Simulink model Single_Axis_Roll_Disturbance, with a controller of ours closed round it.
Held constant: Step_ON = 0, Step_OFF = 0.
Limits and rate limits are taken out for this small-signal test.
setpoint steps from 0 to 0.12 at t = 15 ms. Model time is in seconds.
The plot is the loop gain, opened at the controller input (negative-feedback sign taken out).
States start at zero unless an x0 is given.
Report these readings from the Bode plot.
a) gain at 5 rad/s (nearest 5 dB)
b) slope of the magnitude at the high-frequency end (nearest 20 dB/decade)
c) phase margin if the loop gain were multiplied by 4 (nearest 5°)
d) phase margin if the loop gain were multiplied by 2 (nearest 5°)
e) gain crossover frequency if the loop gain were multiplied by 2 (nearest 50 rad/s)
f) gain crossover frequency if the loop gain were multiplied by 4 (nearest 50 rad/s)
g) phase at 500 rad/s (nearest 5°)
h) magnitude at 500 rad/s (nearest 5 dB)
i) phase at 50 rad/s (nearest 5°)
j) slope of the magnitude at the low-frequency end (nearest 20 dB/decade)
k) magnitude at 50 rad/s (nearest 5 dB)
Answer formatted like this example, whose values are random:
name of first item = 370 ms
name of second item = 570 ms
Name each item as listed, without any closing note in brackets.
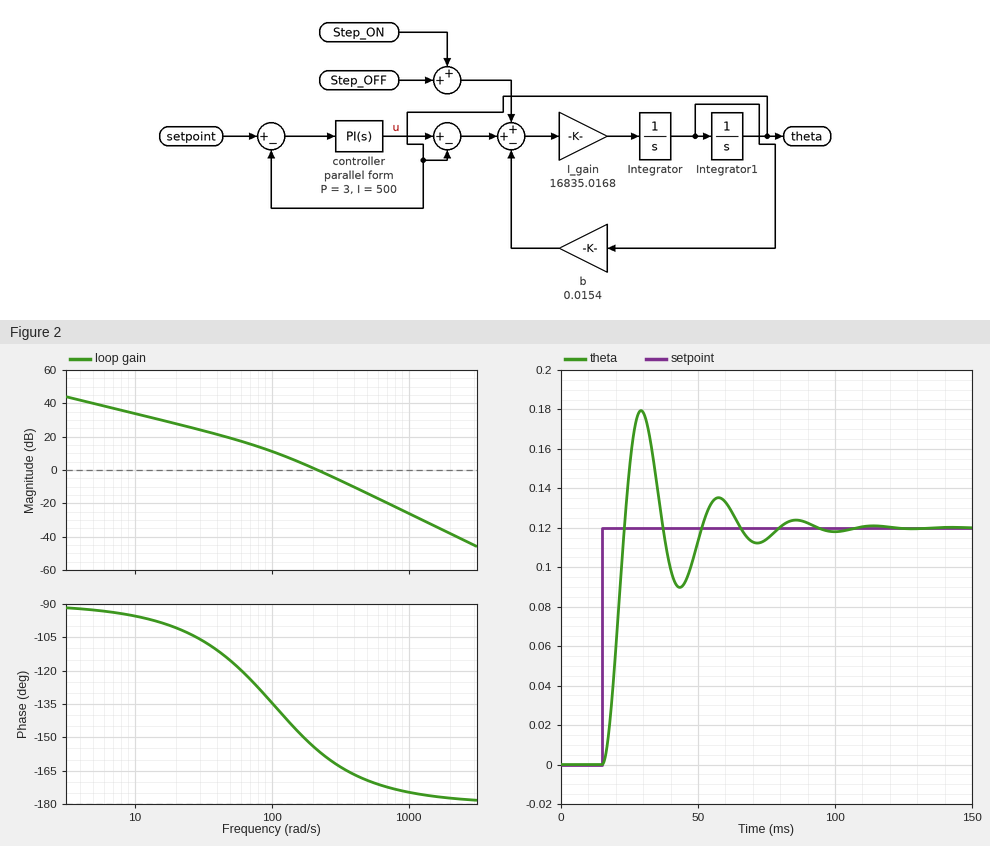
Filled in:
gain at 5 rad/s = 40 dB
slope of the magnitude at the high-frequency end = -40 dB/decade
phase margin if the loop gain were multiplied by 4 = 10°
phase margin if the loop gain were multiplied by 2 = 15°
gain crossover frequency if the loop gain were multiplied by 2 = 300 rad/s
gain crossover frequency if the loop gain were multiplied by 4 = 450 rad/s
phase at 500 rad/s = -170°
magnitude at 500 rad/s = -15 dB
phase at 50 rad/s = -115°
slope of the magnitude at the low-frequency end = -20 dB/decade
magnitude at 50 rad/s = 20 dB
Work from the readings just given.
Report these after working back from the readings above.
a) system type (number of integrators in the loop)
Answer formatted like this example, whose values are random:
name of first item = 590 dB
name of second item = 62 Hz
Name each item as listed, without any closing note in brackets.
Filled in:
system type = 1
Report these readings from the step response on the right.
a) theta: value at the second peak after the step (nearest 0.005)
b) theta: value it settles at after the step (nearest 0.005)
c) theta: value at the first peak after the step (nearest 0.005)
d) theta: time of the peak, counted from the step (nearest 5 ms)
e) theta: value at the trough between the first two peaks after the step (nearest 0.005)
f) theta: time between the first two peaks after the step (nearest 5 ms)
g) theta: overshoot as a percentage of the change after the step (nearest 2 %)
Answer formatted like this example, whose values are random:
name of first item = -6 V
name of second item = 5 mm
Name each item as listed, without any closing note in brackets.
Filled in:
theta: value at the second peak after the step = 0.135
theta: value it settles at after the step = 0.120
theta: value at the first peak after the step = 0.180
theta: time of the peak, counted from the step = 15 ms
theta: value at the trough between the first two peaks after the step = 0.090
theta: time between the first two peaks after the step = 30 ms
theta: overshoot as a percentage of the change after the step = 50 %
